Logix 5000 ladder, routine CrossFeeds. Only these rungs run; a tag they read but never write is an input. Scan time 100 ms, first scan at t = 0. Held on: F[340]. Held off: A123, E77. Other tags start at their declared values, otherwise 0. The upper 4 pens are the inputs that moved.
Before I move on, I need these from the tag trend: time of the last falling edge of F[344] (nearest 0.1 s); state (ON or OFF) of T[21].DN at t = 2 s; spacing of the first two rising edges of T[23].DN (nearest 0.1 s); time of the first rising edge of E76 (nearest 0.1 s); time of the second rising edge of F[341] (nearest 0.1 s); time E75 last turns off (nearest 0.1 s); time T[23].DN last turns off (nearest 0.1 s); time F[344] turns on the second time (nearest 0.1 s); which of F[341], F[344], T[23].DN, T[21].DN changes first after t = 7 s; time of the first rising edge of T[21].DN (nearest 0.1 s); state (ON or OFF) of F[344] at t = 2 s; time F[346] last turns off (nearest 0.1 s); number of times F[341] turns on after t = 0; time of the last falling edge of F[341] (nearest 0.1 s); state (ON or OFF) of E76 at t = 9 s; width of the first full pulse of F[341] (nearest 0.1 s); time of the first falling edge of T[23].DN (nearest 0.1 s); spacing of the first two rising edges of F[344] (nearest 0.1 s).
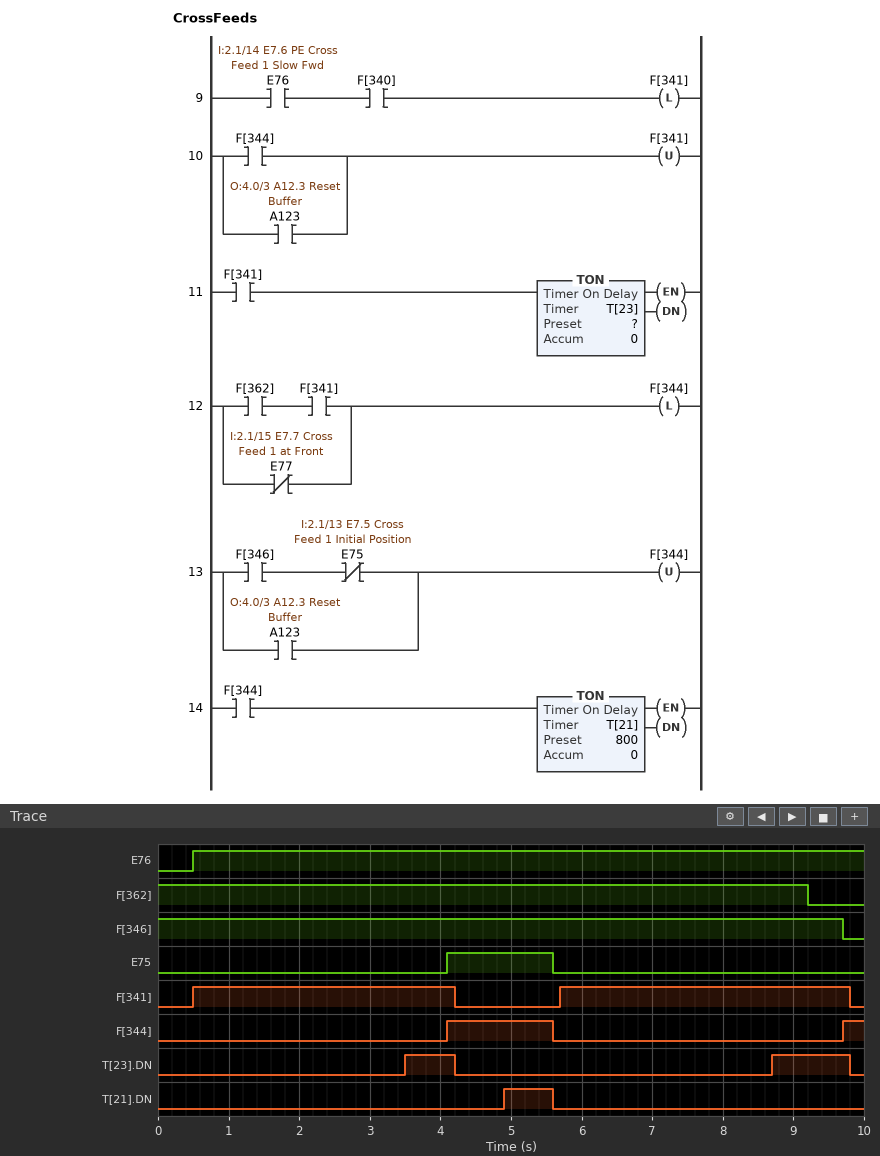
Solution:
5.6 s
OFF
5.2 s
0.5 s
5.7 s
5.6 s
9.8 s
9.7 s
T[23].DN
4.9 s
OFF
9.7 s
2
9.8 s
ON
3.7 s
4.2 s
5.6 s
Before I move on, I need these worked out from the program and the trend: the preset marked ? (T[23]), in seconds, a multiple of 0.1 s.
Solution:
3.0 s
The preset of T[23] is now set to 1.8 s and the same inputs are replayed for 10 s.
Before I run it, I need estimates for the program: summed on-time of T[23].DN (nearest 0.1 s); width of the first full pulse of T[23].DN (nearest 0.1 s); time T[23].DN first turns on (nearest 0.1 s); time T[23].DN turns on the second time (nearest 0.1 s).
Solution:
4.2 s
1.9 s
2.3 s
7.5 s
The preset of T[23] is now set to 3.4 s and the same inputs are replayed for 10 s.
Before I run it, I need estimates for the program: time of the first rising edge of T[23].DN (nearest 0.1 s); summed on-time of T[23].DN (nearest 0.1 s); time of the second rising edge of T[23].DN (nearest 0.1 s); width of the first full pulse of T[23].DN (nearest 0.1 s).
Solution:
3.9 s
1.0 s
9.1 s
0.3 s
